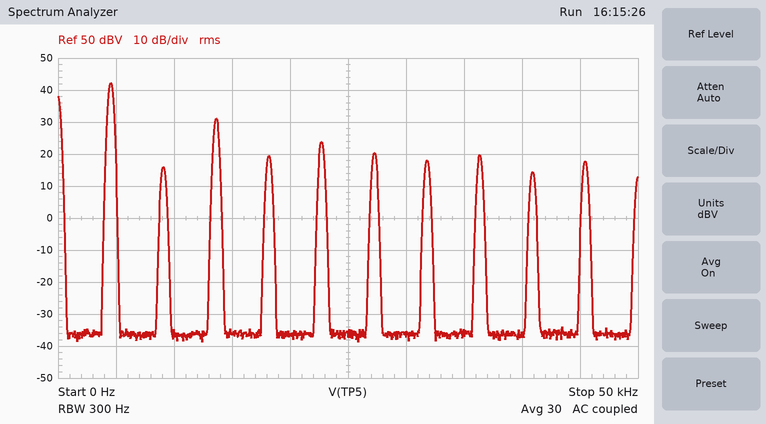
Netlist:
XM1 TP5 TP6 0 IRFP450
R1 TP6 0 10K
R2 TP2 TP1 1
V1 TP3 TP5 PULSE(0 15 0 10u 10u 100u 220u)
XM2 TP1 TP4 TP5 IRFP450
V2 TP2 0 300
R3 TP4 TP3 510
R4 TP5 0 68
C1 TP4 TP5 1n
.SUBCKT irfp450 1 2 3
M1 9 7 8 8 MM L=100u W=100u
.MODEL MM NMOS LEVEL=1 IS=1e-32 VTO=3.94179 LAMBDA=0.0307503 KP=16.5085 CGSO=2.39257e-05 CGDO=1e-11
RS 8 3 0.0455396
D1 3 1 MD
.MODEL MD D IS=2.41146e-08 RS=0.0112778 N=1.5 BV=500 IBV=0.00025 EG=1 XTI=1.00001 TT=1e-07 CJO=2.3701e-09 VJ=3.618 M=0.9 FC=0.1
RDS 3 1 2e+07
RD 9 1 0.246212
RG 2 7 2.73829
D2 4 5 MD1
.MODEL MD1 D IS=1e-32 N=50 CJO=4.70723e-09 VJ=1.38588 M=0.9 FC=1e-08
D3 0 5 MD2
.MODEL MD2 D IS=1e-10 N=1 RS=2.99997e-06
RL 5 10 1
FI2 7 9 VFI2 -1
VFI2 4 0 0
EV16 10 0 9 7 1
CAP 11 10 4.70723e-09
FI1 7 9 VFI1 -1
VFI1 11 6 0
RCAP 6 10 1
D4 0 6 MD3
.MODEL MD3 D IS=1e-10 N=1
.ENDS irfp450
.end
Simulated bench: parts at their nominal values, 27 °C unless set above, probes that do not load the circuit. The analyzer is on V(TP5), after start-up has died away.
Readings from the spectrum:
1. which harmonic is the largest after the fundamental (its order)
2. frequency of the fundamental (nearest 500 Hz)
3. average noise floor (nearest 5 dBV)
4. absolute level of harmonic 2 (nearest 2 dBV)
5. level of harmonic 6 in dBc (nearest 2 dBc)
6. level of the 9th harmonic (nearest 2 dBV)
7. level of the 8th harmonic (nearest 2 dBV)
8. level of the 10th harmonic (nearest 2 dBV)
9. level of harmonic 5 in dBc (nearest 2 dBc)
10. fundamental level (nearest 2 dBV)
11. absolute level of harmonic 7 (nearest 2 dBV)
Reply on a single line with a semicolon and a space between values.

3; 4.5 kHz; -35 dBV; 16 dBV; -22 dBc; 14 dBV; 20 dBV; 18 dBV; -18 dBc; 42 dBV; 18 dBV
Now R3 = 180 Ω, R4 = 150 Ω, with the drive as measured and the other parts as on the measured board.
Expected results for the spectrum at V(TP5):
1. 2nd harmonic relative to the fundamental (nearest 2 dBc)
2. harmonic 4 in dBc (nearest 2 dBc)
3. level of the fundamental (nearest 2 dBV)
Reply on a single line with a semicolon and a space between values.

-20 dBc; -20 dBc; 42 dBV
